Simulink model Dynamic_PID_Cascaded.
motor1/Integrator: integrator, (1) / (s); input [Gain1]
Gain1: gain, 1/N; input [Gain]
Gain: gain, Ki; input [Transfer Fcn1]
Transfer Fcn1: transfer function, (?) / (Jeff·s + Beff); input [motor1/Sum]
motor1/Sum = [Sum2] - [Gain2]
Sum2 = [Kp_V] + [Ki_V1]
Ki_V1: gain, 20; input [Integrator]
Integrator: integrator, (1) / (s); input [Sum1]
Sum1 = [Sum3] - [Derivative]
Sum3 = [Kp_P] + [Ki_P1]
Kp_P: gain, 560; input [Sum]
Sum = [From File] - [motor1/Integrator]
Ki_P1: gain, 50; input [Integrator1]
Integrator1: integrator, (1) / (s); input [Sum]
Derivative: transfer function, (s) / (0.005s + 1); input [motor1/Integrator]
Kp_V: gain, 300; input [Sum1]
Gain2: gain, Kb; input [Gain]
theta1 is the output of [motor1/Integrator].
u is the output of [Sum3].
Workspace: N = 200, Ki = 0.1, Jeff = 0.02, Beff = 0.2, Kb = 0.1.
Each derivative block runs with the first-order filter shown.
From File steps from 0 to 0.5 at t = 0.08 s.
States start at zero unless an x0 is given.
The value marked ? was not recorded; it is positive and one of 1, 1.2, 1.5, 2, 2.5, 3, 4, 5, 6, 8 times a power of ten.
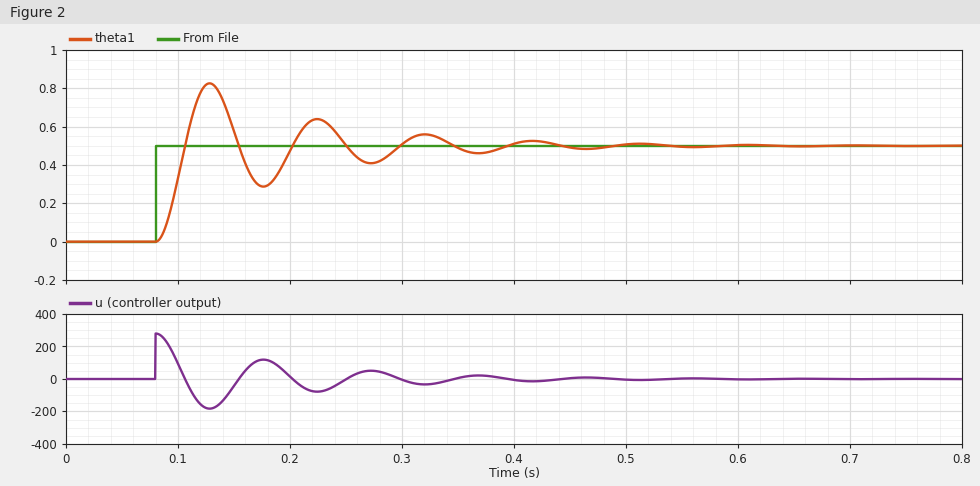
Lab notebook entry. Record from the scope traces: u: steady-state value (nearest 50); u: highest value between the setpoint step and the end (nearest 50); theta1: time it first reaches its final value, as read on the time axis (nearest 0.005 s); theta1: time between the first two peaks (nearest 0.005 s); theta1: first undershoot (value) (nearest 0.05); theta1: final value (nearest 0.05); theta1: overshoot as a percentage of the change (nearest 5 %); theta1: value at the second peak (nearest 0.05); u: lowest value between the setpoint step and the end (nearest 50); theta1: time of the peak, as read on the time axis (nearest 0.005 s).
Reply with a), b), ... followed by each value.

a) 0
b) 300
c) 0.105 s
d) 0.095 s
e) 0.30
f) 0.50
g) 65 %
h) 0.65
i) -200
j) 0.130 s
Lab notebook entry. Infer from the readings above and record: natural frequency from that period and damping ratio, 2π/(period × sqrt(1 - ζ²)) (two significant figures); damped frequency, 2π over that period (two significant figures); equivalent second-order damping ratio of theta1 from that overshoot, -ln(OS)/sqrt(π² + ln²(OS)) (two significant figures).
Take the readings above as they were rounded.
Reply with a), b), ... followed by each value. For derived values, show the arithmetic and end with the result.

a) 2π / (0.095 × sqrt(1 - 0.14²)) = 67 rad/s
b) 2π / 0.095 = 66 rad/s
c) ln(0.65) = -0.431; 0.431 / sqrt(9.870 + 0.186) = 0.14
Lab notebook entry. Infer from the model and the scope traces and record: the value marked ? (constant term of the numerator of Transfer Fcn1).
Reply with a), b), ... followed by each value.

a) 1
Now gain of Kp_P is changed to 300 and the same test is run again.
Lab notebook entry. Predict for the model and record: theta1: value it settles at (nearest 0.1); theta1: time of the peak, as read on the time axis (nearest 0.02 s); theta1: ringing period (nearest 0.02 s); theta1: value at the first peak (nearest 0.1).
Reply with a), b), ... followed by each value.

a) 0.5
b) 0.14 s
c) 0.14 s
d) 0.8
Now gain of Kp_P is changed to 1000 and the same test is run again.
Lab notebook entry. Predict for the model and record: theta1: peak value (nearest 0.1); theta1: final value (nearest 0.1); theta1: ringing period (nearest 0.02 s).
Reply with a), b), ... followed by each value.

a) 0.9
b) 0.5
c) 0.08 s
